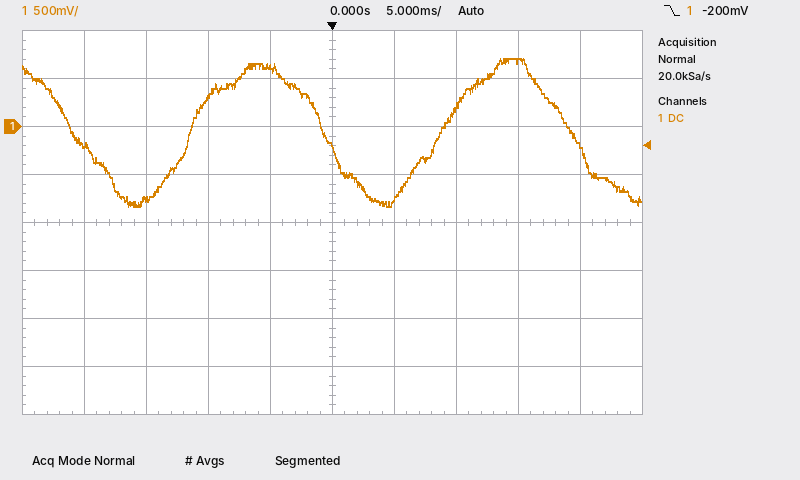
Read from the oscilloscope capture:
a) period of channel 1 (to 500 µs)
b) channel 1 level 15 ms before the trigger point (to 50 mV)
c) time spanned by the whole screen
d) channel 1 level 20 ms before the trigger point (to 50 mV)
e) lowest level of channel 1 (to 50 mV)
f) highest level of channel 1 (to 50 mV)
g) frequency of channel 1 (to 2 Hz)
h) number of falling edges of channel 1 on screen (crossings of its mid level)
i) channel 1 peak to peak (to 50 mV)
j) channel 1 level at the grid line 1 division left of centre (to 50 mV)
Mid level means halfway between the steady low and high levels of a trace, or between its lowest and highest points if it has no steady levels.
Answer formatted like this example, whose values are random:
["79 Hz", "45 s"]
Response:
["20.0 ms", "-750 mV", "50 ms", "-200 mV", "-850 mV", "700 mV", "50 Hz", "3", "1.55 V", "600 mV"]
